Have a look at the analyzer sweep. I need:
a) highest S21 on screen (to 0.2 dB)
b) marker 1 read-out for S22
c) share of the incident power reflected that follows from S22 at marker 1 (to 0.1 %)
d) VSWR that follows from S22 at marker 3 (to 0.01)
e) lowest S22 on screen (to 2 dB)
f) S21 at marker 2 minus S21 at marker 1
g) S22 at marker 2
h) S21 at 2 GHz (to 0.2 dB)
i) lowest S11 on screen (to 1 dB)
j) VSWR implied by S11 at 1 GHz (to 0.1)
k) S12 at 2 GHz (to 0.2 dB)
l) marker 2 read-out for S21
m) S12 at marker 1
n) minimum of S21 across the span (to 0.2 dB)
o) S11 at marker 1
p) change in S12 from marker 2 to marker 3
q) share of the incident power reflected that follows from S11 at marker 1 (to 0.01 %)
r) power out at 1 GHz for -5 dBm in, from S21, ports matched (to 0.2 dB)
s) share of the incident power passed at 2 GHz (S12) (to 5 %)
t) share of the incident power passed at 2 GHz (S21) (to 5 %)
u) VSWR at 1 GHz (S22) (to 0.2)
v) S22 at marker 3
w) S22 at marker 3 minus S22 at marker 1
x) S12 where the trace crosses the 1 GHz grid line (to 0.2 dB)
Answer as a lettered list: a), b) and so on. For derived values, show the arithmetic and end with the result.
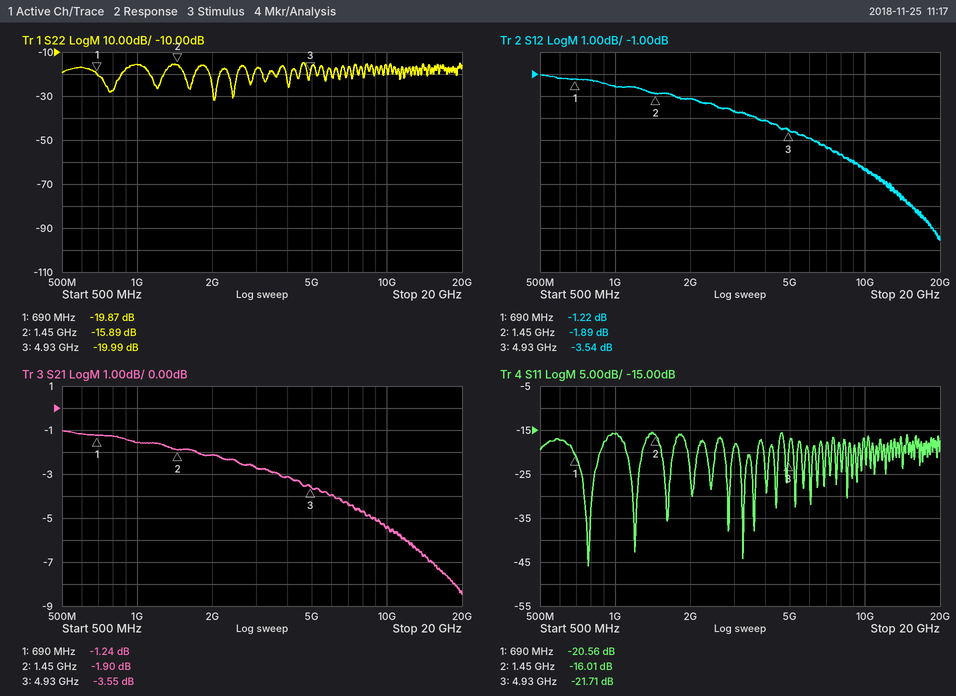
a) -1.0 dB
b) -19.87 dB
c) 10^(-19.87/10) ≈ 1.0 %
d) (1 + 0.1001)/(1 − 0.1001) ≈ 1.22
e) -32 dB
f) -1.9 − (-1.24) = -0.66 dB
g) -15.89 dB
h) -2.2 dB
i) -46 dB
j) |Γ| = 10^(-16/20) = 0.1585; VSWR = (1 + 0.1585)/(1 − 0.1585) ≈ 1.4
k) -2.2 dB
l) -1.90 dB
m) -1.22 dB
n) -8.4 dB
o) -20.56 dB
p) -3.54 − (-1.89) = -1.65 dB
q) 10^(-20.56/10) ≈ 0.88 %
r) -5 dBm + (-1.6 dB) = -6.6 dBm
s) 10^(-2.2/10) ≈ 60 %
t) 10^(-2.2/10) ≈ 60 %
u) |Γ| = 10^(-16/20) = 0.1585; VSWR = (1 + 0.1585)/(1 − 0.1585) ≈ 1.4
v) -19.99 dB
w) -19.99 − (-19.87) = -0.12 dB
x) -1.6 dB
